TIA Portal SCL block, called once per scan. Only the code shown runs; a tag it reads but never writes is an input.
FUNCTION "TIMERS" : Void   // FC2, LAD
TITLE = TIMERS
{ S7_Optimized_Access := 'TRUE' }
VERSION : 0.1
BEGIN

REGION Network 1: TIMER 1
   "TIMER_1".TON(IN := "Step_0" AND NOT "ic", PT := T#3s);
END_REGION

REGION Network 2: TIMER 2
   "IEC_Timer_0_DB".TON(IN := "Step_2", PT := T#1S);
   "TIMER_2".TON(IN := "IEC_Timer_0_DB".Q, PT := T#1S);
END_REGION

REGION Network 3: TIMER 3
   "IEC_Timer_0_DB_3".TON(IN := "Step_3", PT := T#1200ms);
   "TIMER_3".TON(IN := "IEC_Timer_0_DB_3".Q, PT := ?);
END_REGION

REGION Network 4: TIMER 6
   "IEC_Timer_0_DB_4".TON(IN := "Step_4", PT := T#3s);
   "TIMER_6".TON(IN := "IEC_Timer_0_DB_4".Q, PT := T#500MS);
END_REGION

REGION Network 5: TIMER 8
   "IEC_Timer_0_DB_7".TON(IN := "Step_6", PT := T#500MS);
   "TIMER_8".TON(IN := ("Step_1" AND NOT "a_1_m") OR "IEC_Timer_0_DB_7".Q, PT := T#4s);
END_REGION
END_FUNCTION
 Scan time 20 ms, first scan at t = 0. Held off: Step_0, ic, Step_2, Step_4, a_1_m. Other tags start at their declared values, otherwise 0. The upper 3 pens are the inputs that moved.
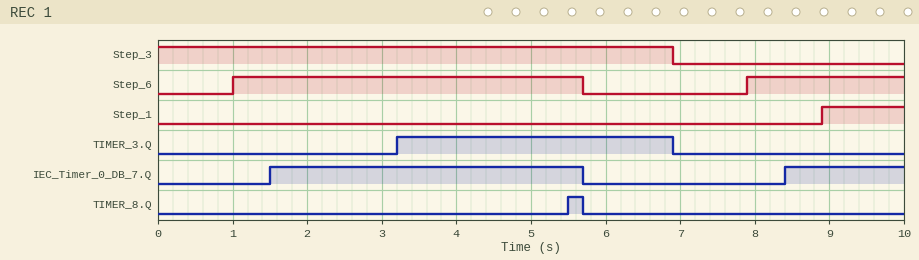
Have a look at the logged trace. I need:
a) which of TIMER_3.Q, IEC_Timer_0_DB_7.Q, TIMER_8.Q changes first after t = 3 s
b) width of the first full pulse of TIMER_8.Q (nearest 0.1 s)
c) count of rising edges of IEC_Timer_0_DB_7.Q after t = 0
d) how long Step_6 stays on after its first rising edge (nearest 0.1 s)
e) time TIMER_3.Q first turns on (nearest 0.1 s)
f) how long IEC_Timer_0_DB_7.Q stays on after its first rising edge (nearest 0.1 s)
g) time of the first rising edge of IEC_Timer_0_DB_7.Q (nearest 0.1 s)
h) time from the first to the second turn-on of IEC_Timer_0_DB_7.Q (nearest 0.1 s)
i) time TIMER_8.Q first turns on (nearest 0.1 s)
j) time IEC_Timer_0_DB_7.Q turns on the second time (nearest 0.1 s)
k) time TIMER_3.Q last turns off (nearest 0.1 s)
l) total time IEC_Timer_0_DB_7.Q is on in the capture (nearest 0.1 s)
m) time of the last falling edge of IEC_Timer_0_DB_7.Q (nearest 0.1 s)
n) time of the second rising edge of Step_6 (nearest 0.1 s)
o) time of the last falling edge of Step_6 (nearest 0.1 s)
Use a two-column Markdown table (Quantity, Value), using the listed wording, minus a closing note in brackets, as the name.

| Quantity | Value |
|---|---|
| which of TIMER_3.Q, IEC_Timer_0_DB_7.Q, TIMER_8.Q changes first after t = 3 s | TIMER_3.Q |
| width of the first full pulse of TIMER_8.Q | 0.2 s |
| count of rising edges of IEC_Timer_0_DB_7.Q after t = 0 | 2 |
| how long Step_6 stays on after its first rising edge | 4.7 s |
| time TIMER_3.Q first turns on | 3.2 s |
| how long IEC_Timer_0_DB_7.Q stays on after its first rising edge | 4.2 s |
| time of the first rising edge of IEC_Timer_0_DB_7.Q | 1.5 s |
| time from the first to the second turn-on of IEC_Timer_0_DB_7.Q | 6.9 s |
| time TIMER_8.Q first turns on | 5.5 s |
| time IEC_Timer_0_DB_7.Q turns on the second time | 8.4 s |
| time TIMER_3.Q last turns off | 6.9 s |
| total time IEC_Timer_0_DB_7.Q is on in the capture | 5.8 s |
| time of the last falling edge of IEC_Timer_0_DB_7.Q | 5.7 s |
| time of the second rising edge of Step_6 | 7.9 s |
| time of the last falling edge of Step_6 | 5.7 s |
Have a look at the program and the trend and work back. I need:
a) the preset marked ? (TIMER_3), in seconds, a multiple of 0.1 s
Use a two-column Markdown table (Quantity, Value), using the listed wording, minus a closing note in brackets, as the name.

| Quantity | Value |
|---|---|
| the preset marked ? (TIMER_3), in seconds, a multiple of 0.1 s | 2.0 s |
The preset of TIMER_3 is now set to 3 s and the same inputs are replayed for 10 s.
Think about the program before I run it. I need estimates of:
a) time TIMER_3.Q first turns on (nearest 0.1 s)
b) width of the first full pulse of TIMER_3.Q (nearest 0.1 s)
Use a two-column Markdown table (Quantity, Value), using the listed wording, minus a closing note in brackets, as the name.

| Quantity | Value |
|---|---|
| time TIMER_3.Q first turns on | 4.2 s |
| width of the first full pulse of TIMER_3.Q | 2.7 s |
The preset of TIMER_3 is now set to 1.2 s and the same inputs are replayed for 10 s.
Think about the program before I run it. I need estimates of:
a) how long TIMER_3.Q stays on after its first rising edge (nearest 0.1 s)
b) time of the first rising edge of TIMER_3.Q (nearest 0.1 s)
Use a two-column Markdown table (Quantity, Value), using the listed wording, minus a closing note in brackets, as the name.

| Quantity | Value |
|---|---|
| how long TIMER_3.Q stays on after its first rising edge | 4.5 s |
| time of the first rising edge of TIMER_3.Q | 2.4 s |
